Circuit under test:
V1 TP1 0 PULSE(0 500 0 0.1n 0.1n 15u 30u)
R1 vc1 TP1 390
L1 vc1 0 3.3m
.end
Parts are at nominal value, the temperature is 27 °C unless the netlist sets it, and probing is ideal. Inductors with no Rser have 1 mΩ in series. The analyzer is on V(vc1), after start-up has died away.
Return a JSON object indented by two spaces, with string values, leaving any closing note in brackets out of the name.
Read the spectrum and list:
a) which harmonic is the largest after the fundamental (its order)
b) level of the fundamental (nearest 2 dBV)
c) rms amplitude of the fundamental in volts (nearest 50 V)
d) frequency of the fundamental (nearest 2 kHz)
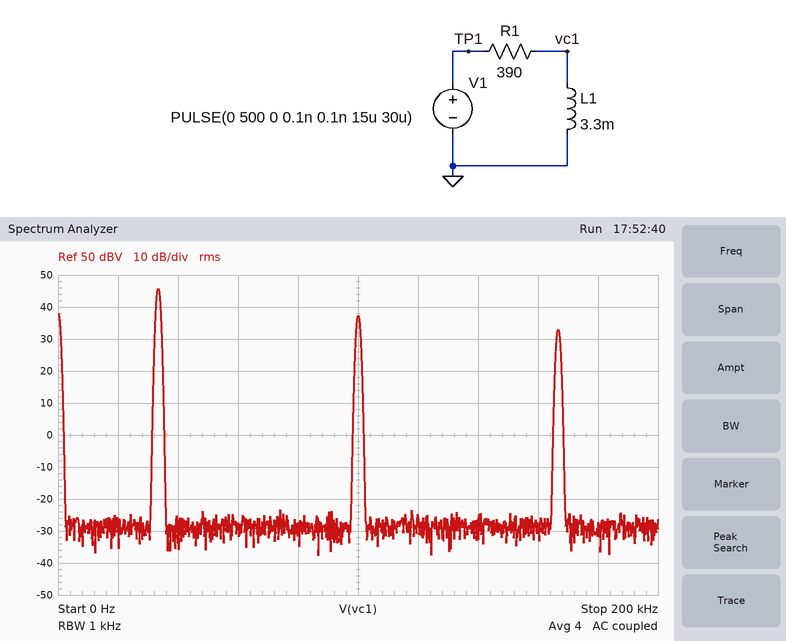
{
  "which harmonic is the largest after the fundamental": "3",
  "level of the fundamental": "46 dBV",
  "rms amplitude of the fundamental in volts": "200 V",
  "frequency of the fundamental": "34 kHz"
}
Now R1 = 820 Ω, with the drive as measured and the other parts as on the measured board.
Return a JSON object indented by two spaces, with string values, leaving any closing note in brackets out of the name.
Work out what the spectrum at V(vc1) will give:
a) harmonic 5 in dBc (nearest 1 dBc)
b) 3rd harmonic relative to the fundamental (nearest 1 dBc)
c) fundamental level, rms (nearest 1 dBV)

{
  "harmonic 5 in dBc": "-10 dBc",
  "3rd harmonic relative to the fundamental": "-6 dBc",
  "fundamental level, rms": "43 dBV"
}
